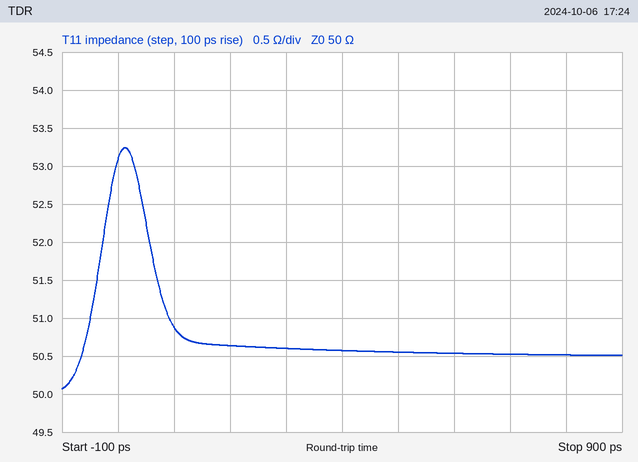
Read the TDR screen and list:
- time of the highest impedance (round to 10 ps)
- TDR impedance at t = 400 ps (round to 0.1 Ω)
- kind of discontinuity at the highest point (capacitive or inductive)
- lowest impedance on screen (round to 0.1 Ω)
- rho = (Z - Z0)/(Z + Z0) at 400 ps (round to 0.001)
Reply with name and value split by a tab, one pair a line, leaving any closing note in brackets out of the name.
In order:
time of the highest impedance	10 ps
TDR impedance at t = 400 ps	50.6 Ω
kind of discontinuity at the highest point	inductive
lowest impedance on screen	50.1 Ω
rho = (Z - Z0)/(Z + Z0) at 400 ps	+0.006
